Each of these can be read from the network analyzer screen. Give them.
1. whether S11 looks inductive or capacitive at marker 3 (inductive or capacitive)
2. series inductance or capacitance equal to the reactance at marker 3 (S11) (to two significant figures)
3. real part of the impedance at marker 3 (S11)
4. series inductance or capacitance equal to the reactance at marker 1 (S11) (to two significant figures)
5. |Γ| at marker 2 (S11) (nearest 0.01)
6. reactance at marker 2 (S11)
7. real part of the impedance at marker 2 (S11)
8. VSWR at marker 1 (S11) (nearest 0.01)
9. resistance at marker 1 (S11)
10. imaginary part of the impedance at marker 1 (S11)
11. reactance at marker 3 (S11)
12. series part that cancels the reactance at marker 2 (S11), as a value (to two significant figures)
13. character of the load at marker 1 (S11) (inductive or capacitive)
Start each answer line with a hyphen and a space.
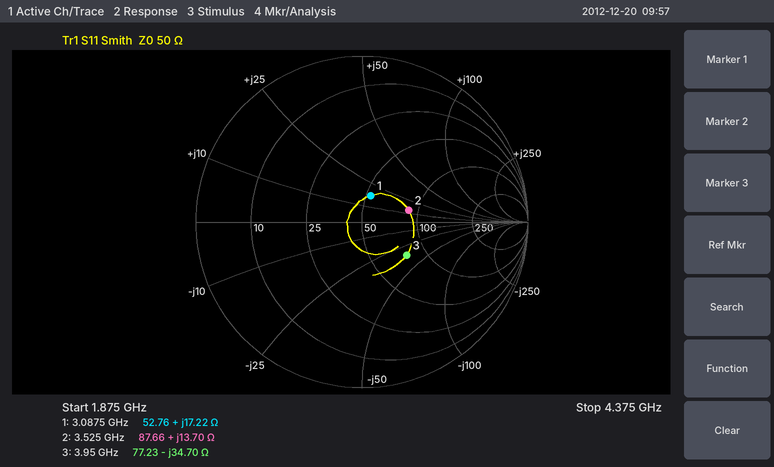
- capacitive
- 1.2 pF
- 77.23 Ω
- 890 pH
- 0.29
- +13.70 Ω
- 87.66 Ω
- 1.40
- 52.76 Ω
- +17.22 Ω
- -34.70 Ω
- 3.3 pF
- inductive
